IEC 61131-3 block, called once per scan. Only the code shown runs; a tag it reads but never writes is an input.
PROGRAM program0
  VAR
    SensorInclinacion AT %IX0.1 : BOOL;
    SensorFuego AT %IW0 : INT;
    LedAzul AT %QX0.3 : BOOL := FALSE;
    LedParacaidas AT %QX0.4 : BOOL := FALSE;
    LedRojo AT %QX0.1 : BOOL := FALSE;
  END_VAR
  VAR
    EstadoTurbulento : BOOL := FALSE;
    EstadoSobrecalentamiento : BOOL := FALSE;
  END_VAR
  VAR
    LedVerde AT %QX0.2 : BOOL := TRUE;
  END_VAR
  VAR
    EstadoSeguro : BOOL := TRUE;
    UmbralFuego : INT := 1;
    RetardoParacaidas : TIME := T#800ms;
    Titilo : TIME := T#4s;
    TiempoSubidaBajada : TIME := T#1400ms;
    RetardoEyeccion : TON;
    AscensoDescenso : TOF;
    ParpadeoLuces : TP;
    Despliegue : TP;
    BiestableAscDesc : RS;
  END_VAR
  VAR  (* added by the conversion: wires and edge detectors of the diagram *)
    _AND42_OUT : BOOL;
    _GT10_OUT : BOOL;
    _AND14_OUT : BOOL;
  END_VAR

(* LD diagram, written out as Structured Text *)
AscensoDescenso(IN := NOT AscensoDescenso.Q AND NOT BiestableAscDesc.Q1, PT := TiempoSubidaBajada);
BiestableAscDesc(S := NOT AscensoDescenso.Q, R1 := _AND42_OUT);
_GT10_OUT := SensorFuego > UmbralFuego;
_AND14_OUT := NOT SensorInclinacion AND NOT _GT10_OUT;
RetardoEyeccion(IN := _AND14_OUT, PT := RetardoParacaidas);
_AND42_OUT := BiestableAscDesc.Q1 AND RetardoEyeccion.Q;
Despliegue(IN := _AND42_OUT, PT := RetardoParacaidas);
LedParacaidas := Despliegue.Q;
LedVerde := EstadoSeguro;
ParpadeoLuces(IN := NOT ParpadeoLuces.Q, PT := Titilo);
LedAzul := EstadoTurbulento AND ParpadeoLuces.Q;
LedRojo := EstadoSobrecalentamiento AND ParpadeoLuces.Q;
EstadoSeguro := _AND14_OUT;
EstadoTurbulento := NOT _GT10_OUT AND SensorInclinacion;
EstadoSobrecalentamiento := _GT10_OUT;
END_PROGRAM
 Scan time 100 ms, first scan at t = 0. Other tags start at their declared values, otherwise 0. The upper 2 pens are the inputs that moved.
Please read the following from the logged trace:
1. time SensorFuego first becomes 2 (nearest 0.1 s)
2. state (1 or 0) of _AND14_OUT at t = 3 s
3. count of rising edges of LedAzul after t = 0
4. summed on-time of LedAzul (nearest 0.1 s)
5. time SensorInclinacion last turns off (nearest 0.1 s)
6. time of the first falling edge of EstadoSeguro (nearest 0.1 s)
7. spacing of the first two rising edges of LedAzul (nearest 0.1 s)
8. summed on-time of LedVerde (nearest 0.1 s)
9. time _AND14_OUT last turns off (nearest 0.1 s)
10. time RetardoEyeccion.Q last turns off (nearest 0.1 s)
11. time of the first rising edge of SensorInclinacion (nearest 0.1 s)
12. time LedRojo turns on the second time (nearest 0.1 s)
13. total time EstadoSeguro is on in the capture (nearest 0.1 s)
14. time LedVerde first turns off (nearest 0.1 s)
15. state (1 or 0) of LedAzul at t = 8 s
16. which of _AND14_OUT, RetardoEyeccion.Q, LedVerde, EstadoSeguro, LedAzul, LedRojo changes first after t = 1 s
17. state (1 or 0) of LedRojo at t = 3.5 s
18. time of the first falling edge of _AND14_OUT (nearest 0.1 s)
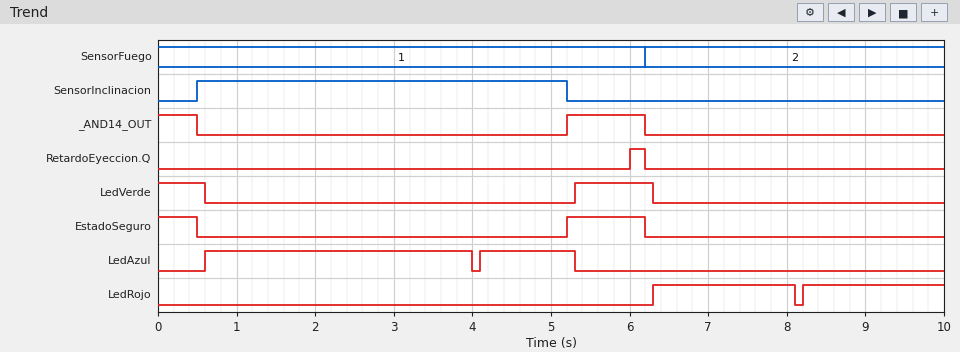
6.2 s
0
2
4.6 s
5.2 s
0.5 s
3.5 s
1.6 s
6.2 s
6.2 s
0.5 s
8.2 s
1.5 s
0.6 s
0
LedAzul
0
0.5 s
